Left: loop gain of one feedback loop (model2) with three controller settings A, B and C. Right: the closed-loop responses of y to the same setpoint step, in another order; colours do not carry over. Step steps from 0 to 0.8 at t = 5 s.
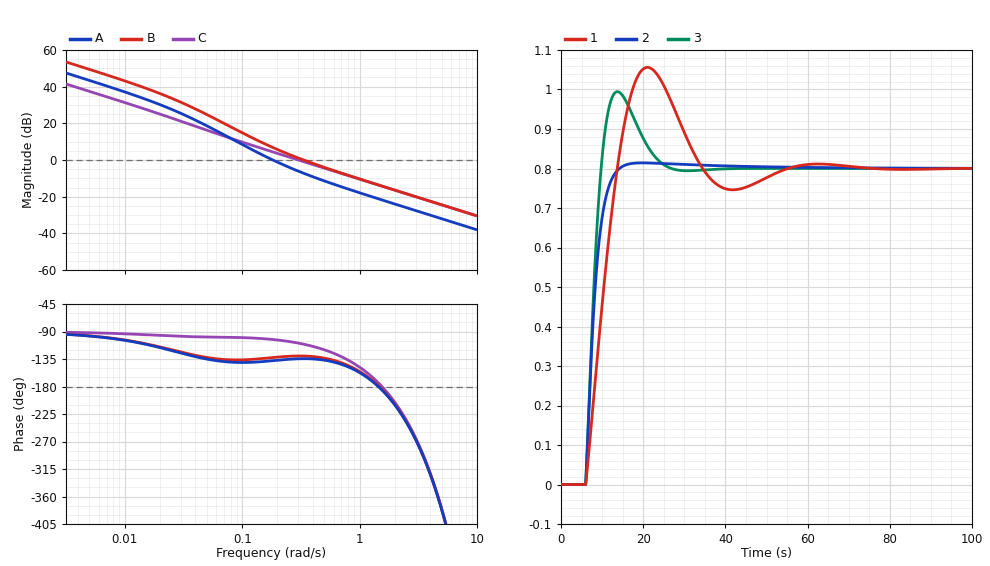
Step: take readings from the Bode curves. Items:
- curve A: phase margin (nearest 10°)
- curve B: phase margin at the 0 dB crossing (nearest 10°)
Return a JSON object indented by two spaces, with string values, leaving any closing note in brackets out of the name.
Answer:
{
  "curve A: phase margin": "40°",
  "curve B: phase margin at the 0 dB crossing": "50°"
}
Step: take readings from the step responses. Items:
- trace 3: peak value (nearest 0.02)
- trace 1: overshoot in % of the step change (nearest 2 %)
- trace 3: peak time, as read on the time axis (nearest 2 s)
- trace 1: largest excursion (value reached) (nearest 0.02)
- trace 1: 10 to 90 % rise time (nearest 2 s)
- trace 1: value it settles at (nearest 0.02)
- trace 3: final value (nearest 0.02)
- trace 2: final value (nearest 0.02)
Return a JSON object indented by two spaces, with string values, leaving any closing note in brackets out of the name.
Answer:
{
  "trace 3: peak value": "1.00",
  "trace 1: overshoot in % of the step change": "32 %",
  "trace 3: peak time, as read on the time axis": "14 s",
  "trace 1: largest excursion (value reached)": "1.06",
  "trace 1: 10 to 90 % rise time": "6 s",
  "trace 1: value it settles at": "0.80",
  "trace 3: final value": "0.80",
  "trace 2: final value": "0.80"
}
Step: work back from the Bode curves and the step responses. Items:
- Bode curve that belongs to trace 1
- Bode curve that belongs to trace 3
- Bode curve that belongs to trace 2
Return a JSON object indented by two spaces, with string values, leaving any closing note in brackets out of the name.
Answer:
{
  "Bode curve that belongs to trace 1": "A",
  "Bode curve that belongs to trace 3": "B",
  "Bode curve that belongs to trace 2": "C"
}
